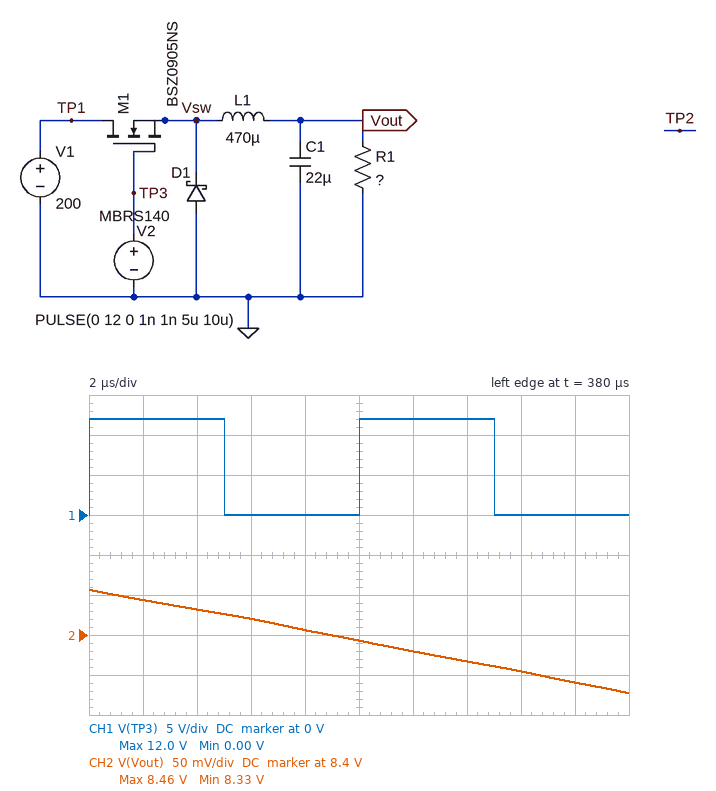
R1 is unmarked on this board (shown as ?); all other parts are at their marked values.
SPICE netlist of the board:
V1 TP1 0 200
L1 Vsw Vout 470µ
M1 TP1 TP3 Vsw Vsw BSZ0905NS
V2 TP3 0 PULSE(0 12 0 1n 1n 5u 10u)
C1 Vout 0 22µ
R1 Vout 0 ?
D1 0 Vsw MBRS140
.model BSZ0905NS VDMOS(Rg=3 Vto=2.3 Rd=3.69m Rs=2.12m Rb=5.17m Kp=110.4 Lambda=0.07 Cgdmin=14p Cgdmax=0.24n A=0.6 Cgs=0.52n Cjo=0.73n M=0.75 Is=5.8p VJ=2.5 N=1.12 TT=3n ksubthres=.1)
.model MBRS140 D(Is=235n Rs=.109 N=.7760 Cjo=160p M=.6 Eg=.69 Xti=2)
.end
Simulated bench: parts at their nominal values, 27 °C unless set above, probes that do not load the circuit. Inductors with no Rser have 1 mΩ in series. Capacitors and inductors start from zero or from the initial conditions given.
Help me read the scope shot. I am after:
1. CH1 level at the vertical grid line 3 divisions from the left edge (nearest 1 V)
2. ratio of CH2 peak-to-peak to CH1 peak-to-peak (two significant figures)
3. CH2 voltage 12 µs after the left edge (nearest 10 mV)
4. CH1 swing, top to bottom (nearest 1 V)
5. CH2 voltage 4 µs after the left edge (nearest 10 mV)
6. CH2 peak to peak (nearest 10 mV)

0 V
0.011
8.38 V
12 V
8.43 V
130 mV
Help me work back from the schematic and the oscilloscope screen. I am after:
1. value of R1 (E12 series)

56 Ω
